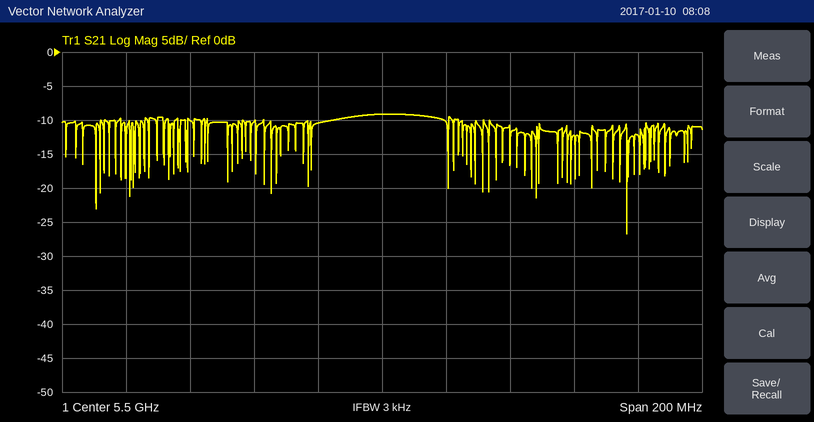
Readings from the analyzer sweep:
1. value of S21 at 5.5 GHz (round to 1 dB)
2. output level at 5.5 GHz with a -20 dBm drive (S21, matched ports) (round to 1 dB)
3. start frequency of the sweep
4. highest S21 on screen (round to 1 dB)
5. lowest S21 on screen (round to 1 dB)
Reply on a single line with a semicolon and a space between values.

-9 dB; -29 dBm; 5.4 GHz; -9 dB; -27 dB
